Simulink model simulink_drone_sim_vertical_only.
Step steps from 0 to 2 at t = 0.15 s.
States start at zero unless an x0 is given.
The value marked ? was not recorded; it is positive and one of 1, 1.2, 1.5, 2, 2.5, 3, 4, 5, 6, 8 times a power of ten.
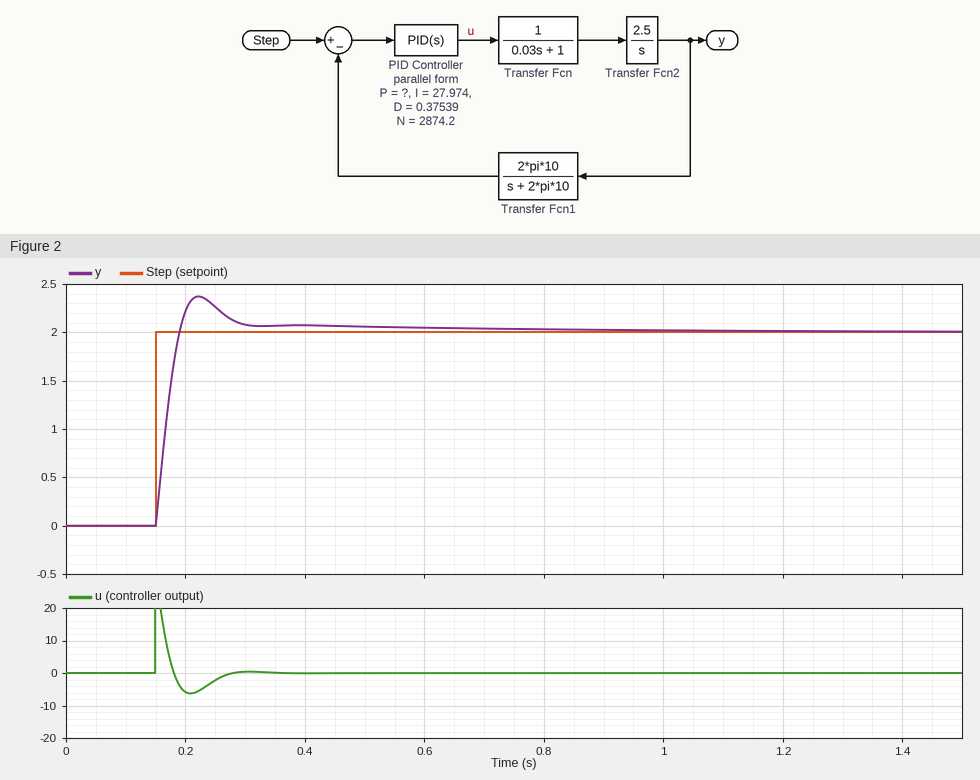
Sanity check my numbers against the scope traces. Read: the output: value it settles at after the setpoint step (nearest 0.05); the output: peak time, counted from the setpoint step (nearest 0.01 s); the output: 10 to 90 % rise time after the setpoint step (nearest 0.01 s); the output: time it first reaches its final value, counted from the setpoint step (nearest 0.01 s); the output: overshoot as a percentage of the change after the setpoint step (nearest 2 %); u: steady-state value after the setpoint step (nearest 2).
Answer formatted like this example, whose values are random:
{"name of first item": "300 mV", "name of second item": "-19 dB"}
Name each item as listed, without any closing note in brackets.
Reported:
{"the output: value it settles at after the setpoint step": "2.00", "the output: peak time, counted from the setpoint step": "0.07 s", "the output: 10 to 90 % rise time after the setpoint step": "0.03 s", "the output: time it first reaches its final value, counted from the setpoint step": "0.04 s", "the output: overshoot as a percentage of the change after the setpoint step": "18 %", "u: steady-state value after the setpoint step": "0"}
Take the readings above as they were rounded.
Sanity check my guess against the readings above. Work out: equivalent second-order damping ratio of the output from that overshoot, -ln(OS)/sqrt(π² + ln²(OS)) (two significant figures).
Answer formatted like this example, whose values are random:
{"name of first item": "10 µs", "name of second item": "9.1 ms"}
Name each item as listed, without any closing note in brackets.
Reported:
{"equivalent second-order damping ratio of the output from that overshoot, -ln(OS)/sqrt(π² + ln²(OS))": "0.48"}
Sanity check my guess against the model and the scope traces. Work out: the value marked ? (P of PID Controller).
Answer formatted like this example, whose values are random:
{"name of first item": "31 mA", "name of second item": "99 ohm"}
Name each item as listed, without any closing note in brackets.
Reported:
{"the value marked ?": "15"}
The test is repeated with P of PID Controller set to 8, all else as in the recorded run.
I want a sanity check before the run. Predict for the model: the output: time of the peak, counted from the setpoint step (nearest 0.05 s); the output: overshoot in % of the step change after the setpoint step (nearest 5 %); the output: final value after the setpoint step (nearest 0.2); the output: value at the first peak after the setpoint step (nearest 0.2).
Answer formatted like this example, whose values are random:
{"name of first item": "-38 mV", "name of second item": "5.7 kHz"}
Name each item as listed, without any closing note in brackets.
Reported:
{"the output: time of the peak, counted from the setpoint step": "0.25 s", "the output: overshoot in % of the step change after the setpoint step": "10 %", "the output: final value after the setpoint step": "2.0", "the output: value at the first peak after the setpoint step": "2.2"}
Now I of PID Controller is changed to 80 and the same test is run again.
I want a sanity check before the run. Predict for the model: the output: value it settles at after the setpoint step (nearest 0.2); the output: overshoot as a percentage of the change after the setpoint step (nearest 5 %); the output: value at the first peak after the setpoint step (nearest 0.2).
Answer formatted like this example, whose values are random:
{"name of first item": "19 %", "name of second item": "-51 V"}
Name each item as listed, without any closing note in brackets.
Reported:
{"the output: value it settles at after the setpoint step": "2.0", "the output: overshoot as a percentage of the change after the setpoint step": "25 %", "the output: value at the first peak after the setpoint step": "2.6"}
